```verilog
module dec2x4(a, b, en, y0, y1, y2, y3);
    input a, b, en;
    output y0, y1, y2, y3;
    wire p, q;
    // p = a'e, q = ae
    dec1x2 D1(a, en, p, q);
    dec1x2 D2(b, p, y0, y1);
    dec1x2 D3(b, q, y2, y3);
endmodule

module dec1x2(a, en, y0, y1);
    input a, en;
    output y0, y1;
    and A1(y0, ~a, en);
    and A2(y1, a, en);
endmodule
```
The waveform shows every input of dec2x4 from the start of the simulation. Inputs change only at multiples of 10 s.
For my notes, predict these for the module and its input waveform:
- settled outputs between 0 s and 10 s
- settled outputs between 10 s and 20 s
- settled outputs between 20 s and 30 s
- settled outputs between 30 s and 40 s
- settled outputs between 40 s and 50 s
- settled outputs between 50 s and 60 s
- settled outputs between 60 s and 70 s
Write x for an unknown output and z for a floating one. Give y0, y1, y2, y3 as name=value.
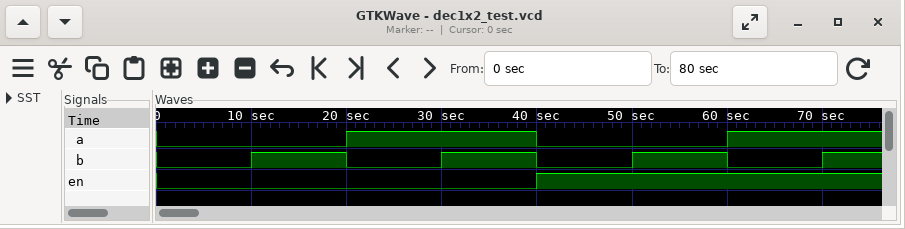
y0=0, y1=0, y2=0, y3=0
y0=0, y1=0, y2=0, y3=0
y0=0, y1=0, y2=0, y3=0
y0=0, y1=0, y2=0, y3=0
y0=1, y1=0, y2=0, y3=0
y0=0, y1=1, y2=0, y3=0
y0=0, y1=0, y2=1, y3=0
